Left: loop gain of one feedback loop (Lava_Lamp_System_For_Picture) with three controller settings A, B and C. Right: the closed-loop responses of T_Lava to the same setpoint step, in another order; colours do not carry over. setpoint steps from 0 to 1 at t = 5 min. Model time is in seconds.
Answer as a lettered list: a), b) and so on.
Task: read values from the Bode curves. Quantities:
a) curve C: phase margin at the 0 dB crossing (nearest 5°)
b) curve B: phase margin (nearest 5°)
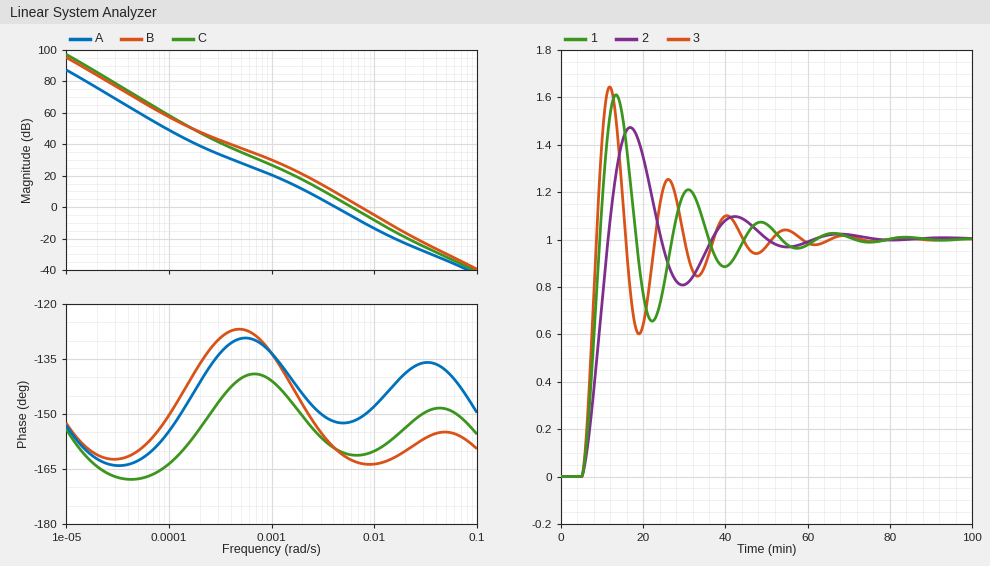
a) 20°
b) 15°
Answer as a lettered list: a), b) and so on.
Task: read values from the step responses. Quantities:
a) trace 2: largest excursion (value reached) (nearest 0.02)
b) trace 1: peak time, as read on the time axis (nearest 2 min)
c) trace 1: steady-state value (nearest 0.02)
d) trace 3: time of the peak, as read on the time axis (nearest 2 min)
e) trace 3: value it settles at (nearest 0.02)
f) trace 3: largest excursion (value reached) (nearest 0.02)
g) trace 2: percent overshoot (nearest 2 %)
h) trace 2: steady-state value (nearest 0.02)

a) 1.48
b) 14 min
c) 1.00
d) 12 min
e) 1.00
f) 1.64
g) 48 %
h) 1.00
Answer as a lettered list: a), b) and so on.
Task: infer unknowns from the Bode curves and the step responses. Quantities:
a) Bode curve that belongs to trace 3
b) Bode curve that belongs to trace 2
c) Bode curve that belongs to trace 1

a) B
b) A
c) C
